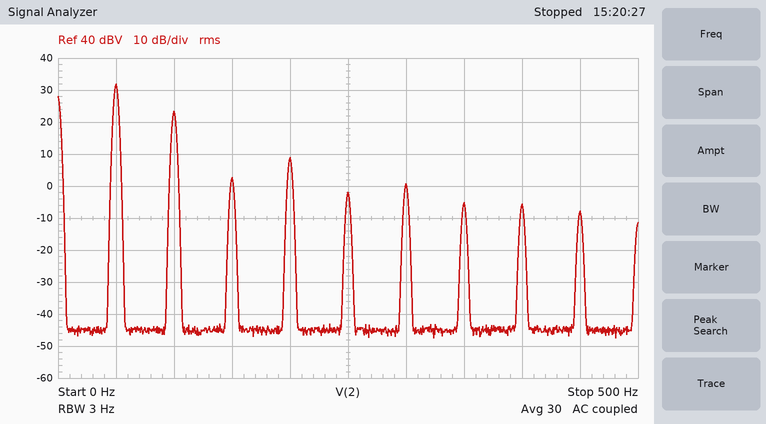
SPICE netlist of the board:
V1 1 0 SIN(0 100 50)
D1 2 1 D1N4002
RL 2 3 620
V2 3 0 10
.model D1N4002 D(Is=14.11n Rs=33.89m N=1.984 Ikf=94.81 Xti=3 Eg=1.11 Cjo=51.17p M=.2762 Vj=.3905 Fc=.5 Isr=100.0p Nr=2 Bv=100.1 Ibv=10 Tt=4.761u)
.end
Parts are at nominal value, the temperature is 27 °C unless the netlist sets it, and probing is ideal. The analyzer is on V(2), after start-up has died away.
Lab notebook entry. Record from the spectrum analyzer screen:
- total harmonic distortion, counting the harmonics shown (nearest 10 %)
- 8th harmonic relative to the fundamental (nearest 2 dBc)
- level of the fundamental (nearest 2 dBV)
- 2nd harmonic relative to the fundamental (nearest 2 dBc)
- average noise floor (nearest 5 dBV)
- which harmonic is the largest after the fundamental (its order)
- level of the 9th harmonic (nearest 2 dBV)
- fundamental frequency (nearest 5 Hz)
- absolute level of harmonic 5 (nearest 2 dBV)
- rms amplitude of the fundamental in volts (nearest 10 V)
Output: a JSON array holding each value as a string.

["40 %", "-38 dBc", "32 dBV", "-8 dBc", "-45 dBV", "2", "-8 dBV", "50 Hz", "-2 dBV", "40 V"]
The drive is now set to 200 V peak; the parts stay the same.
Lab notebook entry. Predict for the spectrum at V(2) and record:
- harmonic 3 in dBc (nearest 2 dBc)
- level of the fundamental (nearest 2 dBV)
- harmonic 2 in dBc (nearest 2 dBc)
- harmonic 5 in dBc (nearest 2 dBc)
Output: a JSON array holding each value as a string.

["-22 dBc", "40 dBV", "-18 dBc", "-50 dBc"]
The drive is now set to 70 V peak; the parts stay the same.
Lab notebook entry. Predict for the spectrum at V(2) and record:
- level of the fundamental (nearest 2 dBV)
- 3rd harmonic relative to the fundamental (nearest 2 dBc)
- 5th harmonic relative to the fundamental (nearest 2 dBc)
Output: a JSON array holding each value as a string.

["30 dBV", "-26 dBc", "-32 dBc"]
